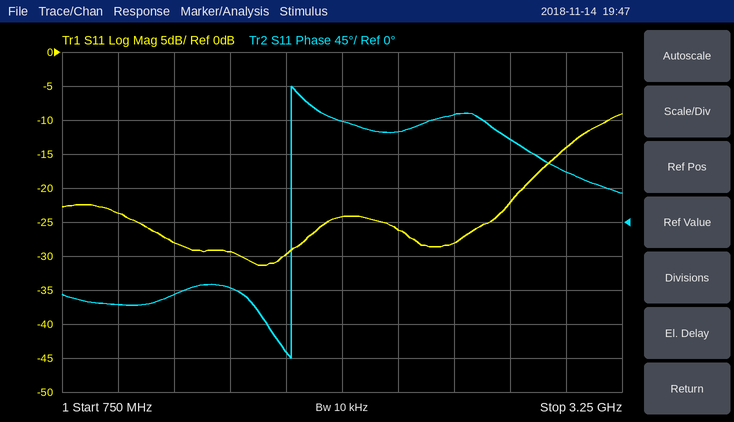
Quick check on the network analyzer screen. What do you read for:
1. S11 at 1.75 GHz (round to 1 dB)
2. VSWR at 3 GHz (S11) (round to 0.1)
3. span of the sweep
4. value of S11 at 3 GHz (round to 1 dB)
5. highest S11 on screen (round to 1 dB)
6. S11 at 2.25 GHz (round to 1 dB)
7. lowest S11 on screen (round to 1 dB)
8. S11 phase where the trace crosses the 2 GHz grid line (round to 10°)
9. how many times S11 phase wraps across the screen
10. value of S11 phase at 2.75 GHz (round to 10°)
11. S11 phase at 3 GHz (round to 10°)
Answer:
-30 dB
1.5
2.5 GHz
-14 dB
-9 dB
-26 dB
-31 dB
130°
1
110°
70°
